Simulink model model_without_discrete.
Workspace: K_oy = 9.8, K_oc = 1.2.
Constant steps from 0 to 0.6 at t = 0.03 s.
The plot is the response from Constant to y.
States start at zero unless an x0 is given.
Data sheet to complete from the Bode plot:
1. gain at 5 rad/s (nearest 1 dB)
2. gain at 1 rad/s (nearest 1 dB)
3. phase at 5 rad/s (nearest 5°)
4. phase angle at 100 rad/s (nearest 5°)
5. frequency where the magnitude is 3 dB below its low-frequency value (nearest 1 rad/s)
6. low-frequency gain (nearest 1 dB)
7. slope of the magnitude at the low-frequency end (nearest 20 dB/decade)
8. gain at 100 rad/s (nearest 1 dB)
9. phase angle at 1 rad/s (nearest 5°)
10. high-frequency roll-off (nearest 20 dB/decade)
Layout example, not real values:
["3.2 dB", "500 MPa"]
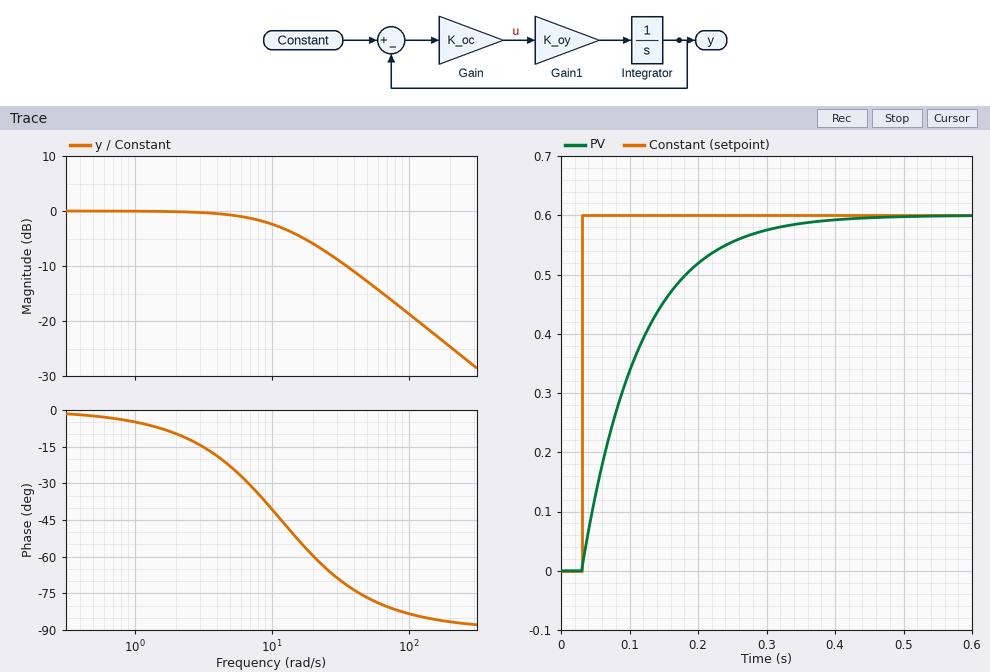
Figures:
["-1 dB", "0 dB", "-25°", "-85°", "12 rad/s", "0 dB", "0 dB/decade", "-19 dB", "-5°", "-20 dB/decade"]
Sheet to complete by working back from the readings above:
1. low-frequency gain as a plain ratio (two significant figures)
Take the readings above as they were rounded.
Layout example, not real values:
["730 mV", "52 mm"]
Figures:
["1.0"]
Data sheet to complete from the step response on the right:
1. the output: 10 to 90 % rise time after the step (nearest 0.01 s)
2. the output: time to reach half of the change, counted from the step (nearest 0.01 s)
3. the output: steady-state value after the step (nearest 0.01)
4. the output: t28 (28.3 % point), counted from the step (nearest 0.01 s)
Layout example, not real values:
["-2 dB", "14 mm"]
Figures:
["0.19 s", "0.06 s", "0.60", "0.03 s"]
